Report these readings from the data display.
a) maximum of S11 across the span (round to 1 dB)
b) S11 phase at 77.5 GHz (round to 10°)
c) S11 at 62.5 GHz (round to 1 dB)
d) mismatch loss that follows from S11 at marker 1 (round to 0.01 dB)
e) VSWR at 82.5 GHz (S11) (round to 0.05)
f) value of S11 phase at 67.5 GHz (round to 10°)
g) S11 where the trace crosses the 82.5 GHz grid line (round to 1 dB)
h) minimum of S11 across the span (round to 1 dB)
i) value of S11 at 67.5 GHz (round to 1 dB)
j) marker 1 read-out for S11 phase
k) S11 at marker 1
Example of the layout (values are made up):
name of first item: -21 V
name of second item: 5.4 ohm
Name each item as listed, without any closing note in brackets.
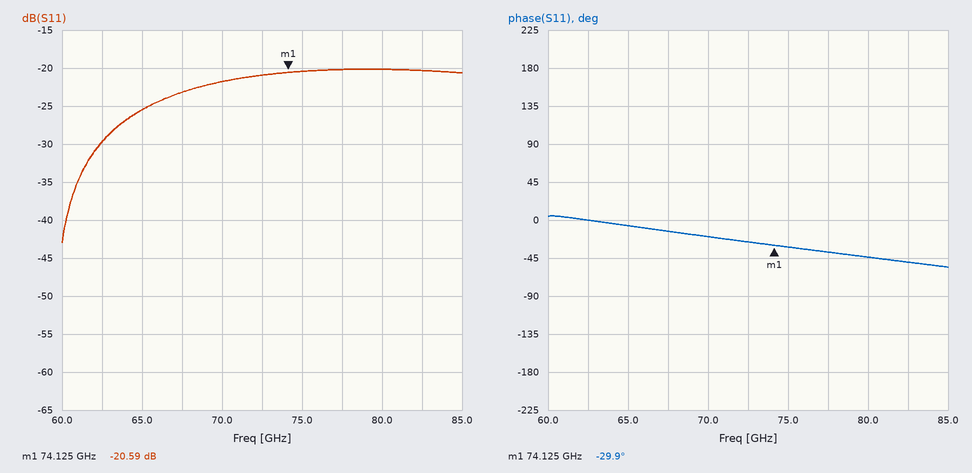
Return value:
maximum of S11 across the span: -20 dB
S11 phase at 77.5 GHz: -40°
S11 at 62.5 GHz: -30 dB
mismatch loss that follows from S11 at marker 1: 0.04 dB
VSWR at 82.5 GHz (S11): 1.20
value of S11 phase at 67.5 GHz: -10°
S11 where the trace crosses the 82.5 GHz grid line: -20 dB
minimum of S11 across the span: -43 dB
value of S11 at 67.5 GHz: -23 dB
marker 1 read-out for S11 phase: -29.9°
S11 at marker 1: -20.59 dB
